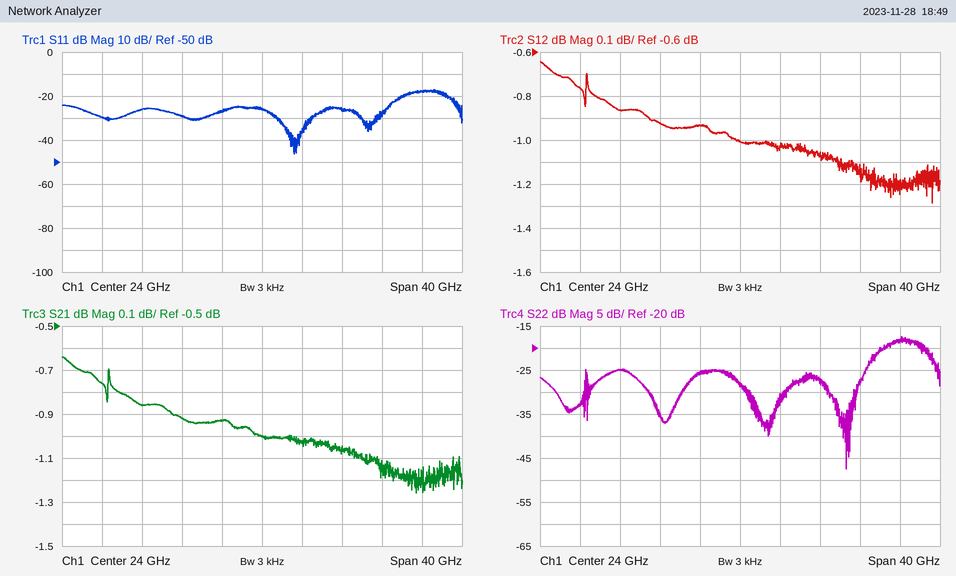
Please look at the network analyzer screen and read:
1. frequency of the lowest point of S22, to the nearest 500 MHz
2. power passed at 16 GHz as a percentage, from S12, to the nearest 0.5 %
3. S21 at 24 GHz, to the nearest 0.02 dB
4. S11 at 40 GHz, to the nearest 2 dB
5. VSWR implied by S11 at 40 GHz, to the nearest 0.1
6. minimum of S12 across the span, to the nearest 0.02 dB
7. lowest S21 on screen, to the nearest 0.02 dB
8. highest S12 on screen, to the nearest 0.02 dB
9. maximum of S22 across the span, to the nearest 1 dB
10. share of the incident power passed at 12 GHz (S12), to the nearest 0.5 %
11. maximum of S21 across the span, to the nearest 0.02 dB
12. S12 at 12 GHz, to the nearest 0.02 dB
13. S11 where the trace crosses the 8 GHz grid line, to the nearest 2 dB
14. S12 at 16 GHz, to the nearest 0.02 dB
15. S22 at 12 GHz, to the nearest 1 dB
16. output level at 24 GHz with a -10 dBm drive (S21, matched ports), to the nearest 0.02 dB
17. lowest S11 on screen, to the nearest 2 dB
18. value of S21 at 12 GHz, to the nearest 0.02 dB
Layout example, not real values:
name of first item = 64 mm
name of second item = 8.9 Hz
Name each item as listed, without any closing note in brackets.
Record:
frequency of the lowest point of S22, to the nearest 500 MHz = 34.5 GHz
power passed at 16 GHz as a percentage, from S12, to the nearest 0.5 % = 81.0 %
S21 at 24 GHz, to the nearest 0.02 dB = -1.00 dB
S11 at 40 GHz, to the nearest 2 dB = -18 dB
VSWR implied by S11 at 40 GHz, to the nearest 0.1 = 1.3
minimum of S12 across the span, to the nearest 0.02 dB = -1.28 dB
lowest S21 on screen, to the nearest 0.02 dB = -1.26 dB
highest S12 on screen, to the nearest 0.02 dB = -0.64 dB
maximum of S22 across the span, to the nearest 1 dB = -17 dB
share of the incident power passed at 12 GHz (S12), to the nearest 0.5 % = 82.0 %
maximum of S21 across the span, to the nearest 0.02 dB = -0.64 dB
S12 at 12 GHz, to the nearest 0.02 dB = -0.86 dB
S11 where the trace crosses the 8 GHz grid line, to the nearest 2 dB = -30 dB
S12 at 16 GHz, to the nearest 0.02 dB = -0.92 dB
S22 at 12 GHz, to the nearest 1 dB = -25 dB
output level at 24 GHz with a -10 dBm drive (S21, matched ports), to the nearest 0.02 dB = -11.00 dBm
lowest S11 on screen, to the nearest 2 dB = -46 dB
value of S21 at 12 GHz, to the nearest 0.02 dB = -0.86 dB
